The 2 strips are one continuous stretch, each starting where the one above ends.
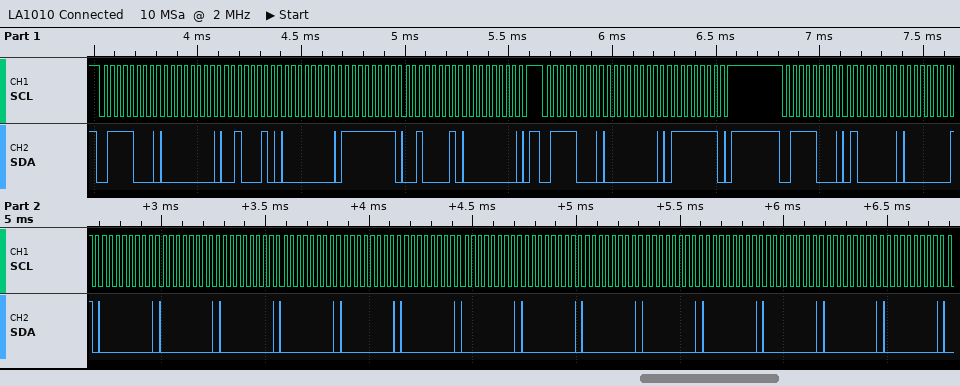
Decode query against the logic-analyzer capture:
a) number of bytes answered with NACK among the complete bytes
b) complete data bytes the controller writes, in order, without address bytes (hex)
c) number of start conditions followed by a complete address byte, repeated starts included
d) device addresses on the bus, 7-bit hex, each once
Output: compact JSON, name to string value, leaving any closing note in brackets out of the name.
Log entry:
{"number of bytes answered with NACK among the complete bytes": "0", "complete data bytes the controller writes, in order, without address bytes": "00 22 00 FF 21 00 00 7F 40 01 00 00 00 00 00 00 00 00 00 00 00 00 00 00", "number of start conditions followed by a complete address byte, repeated starts included": "3", "device addresses on the bus, 7-bit hex, each once": "0x3C"}
